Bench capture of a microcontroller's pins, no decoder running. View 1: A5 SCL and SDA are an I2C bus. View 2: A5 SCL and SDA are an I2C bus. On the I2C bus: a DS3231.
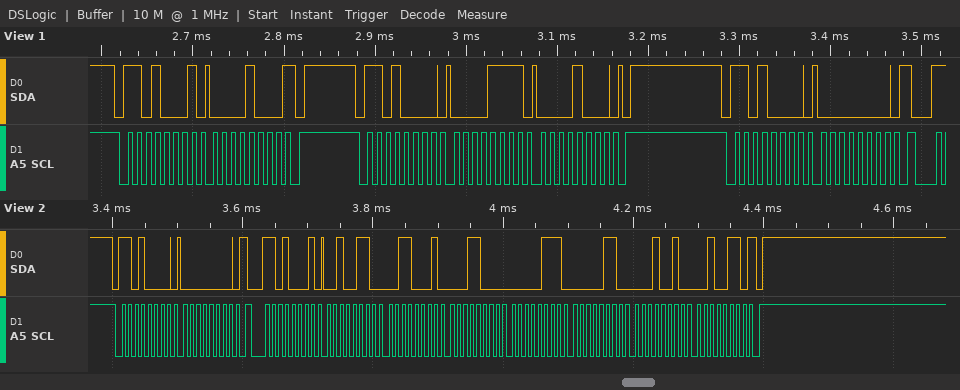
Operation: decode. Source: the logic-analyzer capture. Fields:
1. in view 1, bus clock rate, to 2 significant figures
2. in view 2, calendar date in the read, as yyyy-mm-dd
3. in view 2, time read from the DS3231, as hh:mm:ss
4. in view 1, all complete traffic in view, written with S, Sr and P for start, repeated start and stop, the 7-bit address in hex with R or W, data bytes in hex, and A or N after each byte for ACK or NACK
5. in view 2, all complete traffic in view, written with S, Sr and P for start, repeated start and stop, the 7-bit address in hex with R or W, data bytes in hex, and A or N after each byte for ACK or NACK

100 kHz
2026-12-06
18:31:26
S 68R A 08 N P S 68W A 0F A 08 A P S 68W A 00 A
S 68W A 00 A Sr 68R A 26 A 31 A 18 A 07 A 06 A 12 A 26 N P
